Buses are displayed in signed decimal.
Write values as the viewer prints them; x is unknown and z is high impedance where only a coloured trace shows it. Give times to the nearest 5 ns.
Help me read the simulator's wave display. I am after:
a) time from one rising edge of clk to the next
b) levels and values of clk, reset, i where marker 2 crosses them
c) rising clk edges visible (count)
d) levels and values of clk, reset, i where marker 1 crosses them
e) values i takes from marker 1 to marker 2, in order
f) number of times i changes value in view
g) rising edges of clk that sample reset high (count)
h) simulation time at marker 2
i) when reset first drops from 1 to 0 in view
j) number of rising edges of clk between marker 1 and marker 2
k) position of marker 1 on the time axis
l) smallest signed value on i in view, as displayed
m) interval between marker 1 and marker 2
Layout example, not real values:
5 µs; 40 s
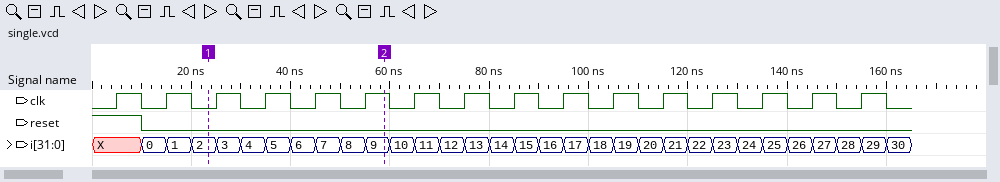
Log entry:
10 ns; clk=1, reset=0, i=9; 16; clk=0, reset=0, i=2; 2, 3, 4, 5, 6, 7, 8, 9; 31; 1; 60 ns; 10 ns; 4; 25 ns; 0; 35 ns
